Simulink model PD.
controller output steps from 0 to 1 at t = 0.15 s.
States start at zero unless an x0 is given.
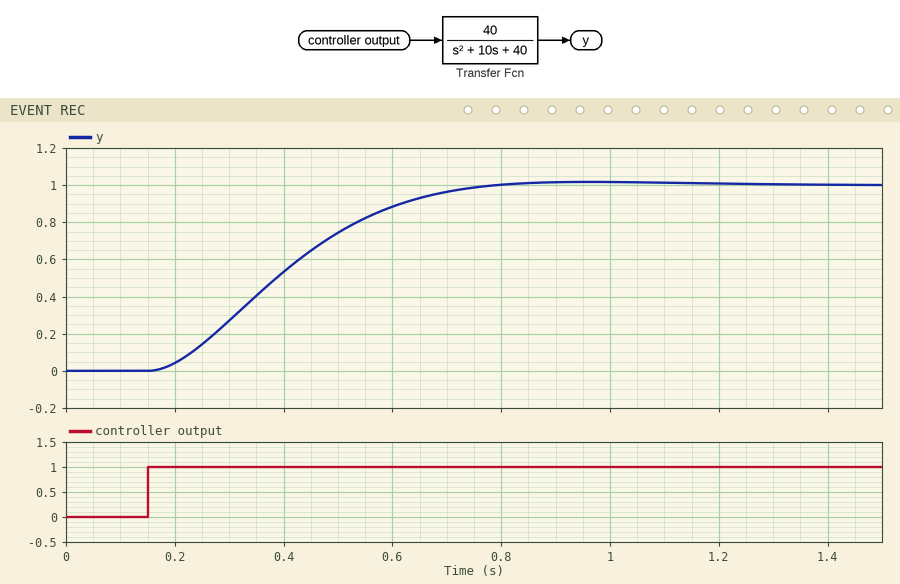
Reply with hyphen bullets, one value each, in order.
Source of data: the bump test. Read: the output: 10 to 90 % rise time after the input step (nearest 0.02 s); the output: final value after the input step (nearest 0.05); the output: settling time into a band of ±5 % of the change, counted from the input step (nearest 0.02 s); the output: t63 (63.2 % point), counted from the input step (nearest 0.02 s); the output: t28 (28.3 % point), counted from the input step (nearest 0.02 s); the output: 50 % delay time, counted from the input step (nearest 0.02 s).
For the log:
- 0.38 s
- 1.00
- 0.52 s
- 0.30 s
- 0.16 s
- 0.24 s
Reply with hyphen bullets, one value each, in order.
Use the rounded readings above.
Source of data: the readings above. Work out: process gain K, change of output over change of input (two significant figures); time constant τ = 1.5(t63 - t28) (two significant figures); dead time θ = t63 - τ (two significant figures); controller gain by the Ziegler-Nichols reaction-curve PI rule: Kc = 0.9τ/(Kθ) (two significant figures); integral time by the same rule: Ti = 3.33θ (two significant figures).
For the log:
- 1.0
- 0.21 s
- 0.090 s
- 2.1
- 0.30 s
